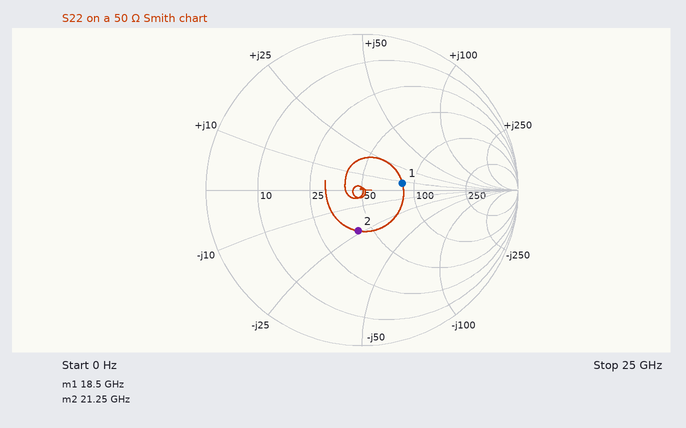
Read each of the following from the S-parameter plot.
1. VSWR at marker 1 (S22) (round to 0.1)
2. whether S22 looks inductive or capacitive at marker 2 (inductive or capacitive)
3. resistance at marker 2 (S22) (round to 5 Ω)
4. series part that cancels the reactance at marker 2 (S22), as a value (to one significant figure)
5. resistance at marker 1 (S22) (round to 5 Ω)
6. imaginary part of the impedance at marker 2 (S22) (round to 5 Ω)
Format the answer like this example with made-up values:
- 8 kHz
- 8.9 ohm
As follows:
- 1.7
- capacitive
- 40 Ω
- 200 pH
- 85 Ω
- -25 Ω
